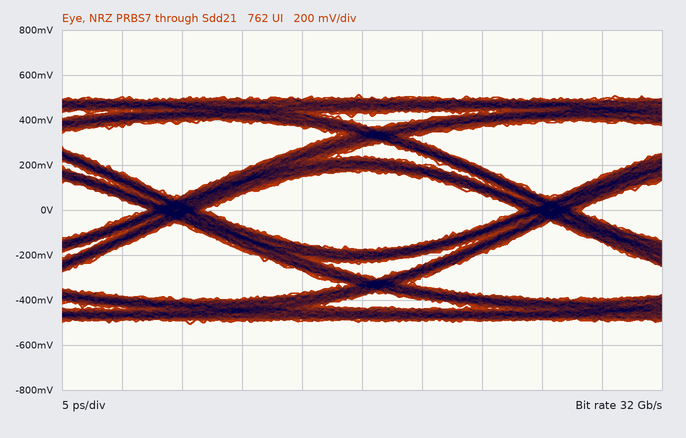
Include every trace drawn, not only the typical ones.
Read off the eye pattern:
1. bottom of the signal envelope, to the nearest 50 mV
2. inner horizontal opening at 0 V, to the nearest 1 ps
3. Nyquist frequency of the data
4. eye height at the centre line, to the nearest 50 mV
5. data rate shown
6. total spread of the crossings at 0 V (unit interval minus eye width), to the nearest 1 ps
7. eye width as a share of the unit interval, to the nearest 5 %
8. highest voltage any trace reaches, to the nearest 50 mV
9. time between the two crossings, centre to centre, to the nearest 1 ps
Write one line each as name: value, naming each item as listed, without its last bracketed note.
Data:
bottom of the signal envelope, to the nearest 50 mV: -500 mV
inner horizontal opening at 0 V, to the nearest 1 ps: 26 ps
Nyquist frequency of the data: 16 GHz
eye height at the centre line, to the nearest 50 mV: 350 mV
data rate shown: 32 Gb/s
total spread of the crossings at 0 V (unit interval minus eye width), to the nearest 1 ps: 5 ps
eye width as a share of the unit interval, to the nearest 5 %: 85 %
highest voltage any trace reaches, to the nearest 50 mV: 500 mV
time between the two crossings, centre to centre, to the nearest 1 ps: 31 ps
